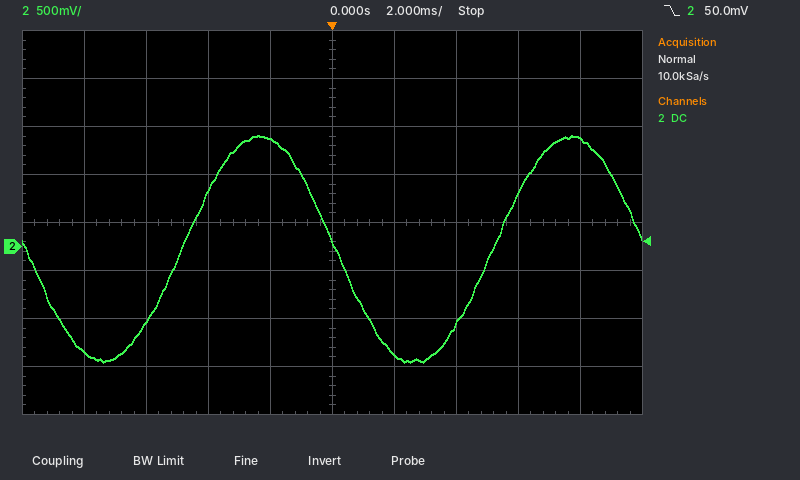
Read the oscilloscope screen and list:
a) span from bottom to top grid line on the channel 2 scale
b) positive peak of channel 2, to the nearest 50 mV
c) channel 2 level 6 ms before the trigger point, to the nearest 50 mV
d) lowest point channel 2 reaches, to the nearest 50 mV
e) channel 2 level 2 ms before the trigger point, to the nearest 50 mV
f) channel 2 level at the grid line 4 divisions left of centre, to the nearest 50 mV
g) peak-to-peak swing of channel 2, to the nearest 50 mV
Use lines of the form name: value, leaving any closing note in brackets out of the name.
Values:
span from bottom to top grid line on the channel 2 scale: 4 V
positive peak of channel 2, to the nearest 50 mV: 1.15 V
channel 2 level 6 ms before the trigger point, to the nearest 50 mV: -800 mV
lowest point channel 2 reaches, to the nearest 50 mV: -1.20 V
channel 2 level 2 ms before the trigger point, to the nearest 50 mV: 1.10 V
channel 2 level at the grid line 4 divisions left of centre, to the nearest 50 mV: -1.10 V
peak-to-peak swing of channel 2, to the nearest 50 mV: 2.35 V
